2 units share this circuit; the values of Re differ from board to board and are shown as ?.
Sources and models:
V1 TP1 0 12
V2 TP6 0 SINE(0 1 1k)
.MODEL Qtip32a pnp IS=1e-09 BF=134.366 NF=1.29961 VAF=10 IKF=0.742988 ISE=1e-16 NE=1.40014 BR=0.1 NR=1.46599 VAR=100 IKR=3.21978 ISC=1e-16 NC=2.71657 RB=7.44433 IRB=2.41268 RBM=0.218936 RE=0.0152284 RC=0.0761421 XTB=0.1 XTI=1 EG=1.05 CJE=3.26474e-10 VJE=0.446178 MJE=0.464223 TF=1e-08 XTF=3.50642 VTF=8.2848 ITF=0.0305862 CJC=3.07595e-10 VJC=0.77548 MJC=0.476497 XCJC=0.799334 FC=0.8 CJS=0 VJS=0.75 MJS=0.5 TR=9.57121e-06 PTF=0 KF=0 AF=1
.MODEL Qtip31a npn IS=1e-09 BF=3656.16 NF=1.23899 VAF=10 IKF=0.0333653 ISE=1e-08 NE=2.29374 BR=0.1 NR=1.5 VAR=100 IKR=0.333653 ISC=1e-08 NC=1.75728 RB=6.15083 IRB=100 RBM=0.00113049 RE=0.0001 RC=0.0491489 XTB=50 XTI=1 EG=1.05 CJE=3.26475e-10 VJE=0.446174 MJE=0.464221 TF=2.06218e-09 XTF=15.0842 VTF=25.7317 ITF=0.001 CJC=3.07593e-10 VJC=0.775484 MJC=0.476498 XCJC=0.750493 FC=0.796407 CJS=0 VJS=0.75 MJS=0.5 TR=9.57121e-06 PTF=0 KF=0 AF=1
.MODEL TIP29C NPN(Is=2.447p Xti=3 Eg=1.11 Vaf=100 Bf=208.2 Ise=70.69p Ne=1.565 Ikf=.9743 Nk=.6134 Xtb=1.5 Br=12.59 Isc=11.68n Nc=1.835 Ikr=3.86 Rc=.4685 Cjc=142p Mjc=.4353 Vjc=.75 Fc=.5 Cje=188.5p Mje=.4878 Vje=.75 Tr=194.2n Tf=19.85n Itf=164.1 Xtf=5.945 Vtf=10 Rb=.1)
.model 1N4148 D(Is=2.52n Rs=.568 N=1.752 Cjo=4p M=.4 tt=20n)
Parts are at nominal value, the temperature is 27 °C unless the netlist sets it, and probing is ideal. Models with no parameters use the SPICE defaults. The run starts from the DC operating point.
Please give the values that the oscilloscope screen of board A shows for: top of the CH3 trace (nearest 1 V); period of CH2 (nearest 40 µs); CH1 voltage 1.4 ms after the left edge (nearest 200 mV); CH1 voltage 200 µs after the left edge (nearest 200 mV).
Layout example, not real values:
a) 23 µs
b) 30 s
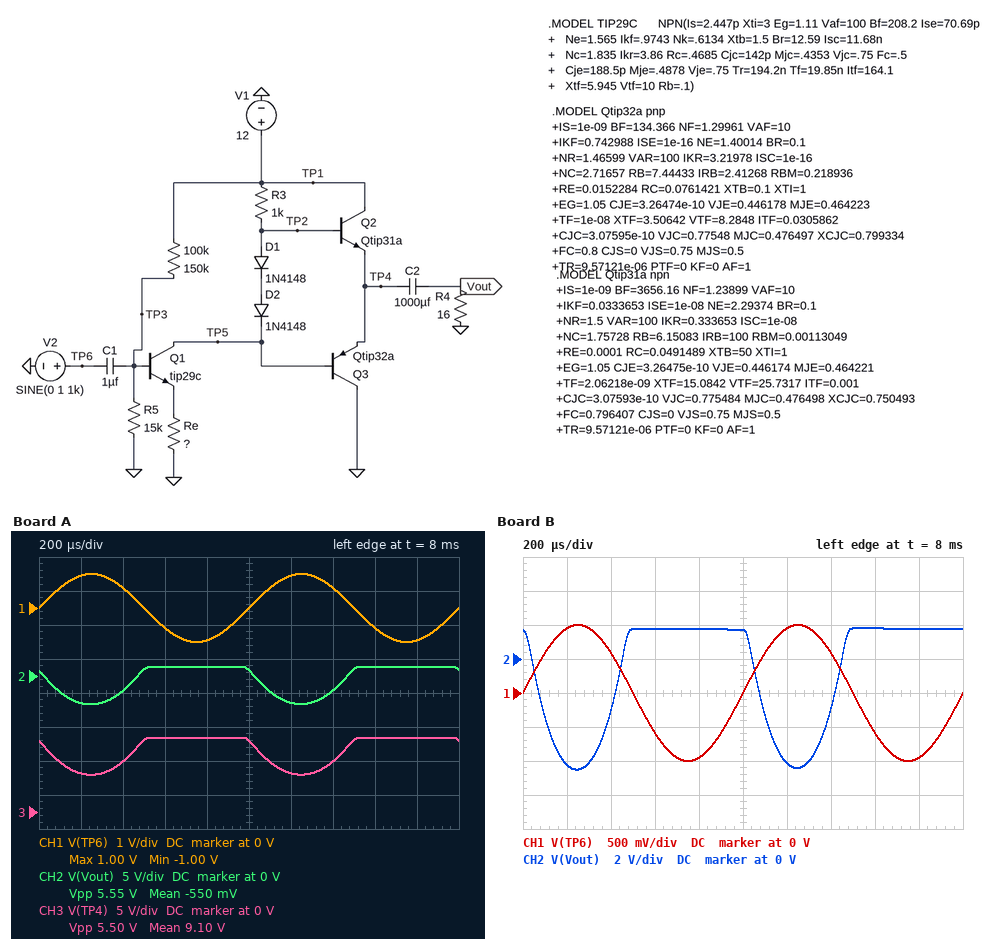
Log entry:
a) 11 V
b) 1.00 ms
c) 600 mV
d) 1.0 V
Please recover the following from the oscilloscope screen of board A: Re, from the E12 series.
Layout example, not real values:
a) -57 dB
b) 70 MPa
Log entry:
a) 120 Ω
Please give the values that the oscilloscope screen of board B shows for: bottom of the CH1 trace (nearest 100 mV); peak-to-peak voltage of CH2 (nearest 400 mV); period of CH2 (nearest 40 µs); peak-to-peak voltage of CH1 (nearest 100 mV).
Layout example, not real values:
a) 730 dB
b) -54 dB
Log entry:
a) -1.0 V
b) 8.4 V
c) 1.00 ms
d) 2.0 V
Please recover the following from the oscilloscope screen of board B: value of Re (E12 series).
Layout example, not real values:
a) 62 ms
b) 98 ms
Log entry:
a) 56 Ω
